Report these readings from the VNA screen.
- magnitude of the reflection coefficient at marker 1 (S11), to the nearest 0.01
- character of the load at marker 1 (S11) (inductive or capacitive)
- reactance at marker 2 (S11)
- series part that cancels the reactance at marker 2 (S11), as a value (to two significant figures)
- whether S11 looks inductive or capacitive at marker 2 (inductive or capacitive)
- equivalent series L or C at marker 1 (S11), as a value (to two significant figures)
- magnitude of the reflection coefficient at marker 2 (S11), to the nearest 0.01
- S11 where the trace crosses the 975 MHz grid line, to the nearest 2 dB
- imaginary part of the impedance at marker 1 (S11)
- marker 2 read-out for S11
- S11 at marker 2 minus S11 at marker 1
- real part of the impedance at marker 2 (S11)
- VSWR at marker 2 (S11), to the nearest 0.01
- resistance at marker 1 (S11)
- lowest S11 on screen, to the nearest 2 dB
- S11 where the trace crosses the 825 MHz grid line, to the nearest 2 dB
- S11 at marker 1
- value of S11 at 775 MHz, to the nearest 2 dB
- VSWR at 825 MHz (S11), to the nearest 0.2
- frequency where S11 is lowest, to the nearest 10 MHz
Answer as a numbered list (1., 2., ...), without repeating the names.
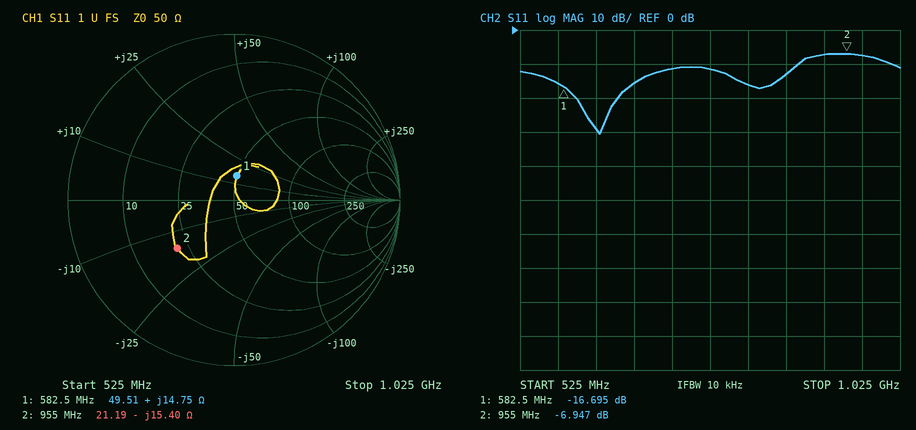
1. 0.15
2. inductive
3. -15.40 Ω
4. 2.6 nH
5. capacitive
6. 4.0 nH
7. 0.45
8. -8 dB
9. +14.75 Ω
10. -6.947 dB
11. 9.748 dB
12. 21.19 Ω
13. 2.63
14. 49.51 Ω
15. -30 dB
16. -16 dB
17. -16.695 dB
18. -12 dB
19. 1.4
20. 630 MHz
